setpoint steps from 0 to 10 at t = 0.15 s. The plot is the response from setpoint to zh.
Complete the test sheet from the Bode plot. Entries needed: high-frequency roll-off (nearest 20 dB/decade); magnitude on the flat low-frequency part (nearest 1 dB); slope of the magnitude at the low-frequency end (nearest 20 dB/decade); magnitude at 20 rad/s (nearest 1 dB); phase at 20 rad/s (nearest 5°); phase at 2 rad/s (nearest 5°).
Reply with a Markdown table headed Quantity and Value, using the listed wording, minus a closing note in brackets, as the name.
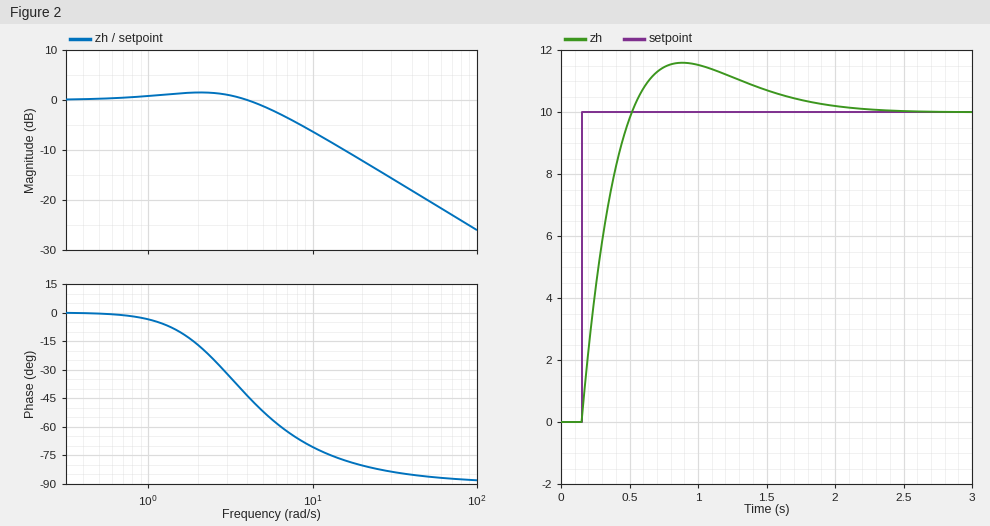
| Quantity | Value |
|---|---|
| high-frequency roll-off | -20 dB/decade |
| magnitude on the flat low-frequency part | 0 dB |
| slope of the magnitude at the low-frequency end | 0 dB/decade |
| magnitude at 20 rad/s | -12 dB |
| phase at 20 rad/s | -80° |
| phase at 2 rad/s | -15° |
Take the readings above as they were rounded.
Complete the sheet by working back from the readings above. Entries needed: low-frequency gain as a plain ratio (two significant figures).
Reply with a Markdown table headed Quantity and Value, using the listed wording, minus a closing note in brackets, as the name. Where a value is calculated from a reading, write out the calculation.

| Quantity | Value |
|---|---|
| low-frequency gain as a plain ratio | 10^(0 / 20) = 1.0 |
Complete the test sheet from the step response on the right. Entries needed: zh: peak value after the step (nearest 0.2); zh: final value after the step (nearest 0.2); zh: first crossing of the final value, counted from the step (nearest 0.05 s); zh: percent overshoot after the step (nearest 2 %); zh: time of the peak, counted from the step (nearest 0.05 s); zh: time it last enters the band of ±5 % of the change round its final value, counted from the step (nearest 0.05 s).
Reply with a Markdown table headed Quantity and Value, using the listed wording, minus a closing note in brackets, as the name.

| Quantity | Value |
|---|---|
| zh: peak value after the step | 11.6 |
| zh: final value after the step | 10.0 |
| zh: first crossing of the final value, counted from the step | 0.35 s |
| zh: percent overshoot after the step | 16 % |
| zh: time of the peak, counted from the step | 0.75 s |
| zh: time it last enters the band of ±5 % of the change round its final value, counted from the step | 1.50 s |
